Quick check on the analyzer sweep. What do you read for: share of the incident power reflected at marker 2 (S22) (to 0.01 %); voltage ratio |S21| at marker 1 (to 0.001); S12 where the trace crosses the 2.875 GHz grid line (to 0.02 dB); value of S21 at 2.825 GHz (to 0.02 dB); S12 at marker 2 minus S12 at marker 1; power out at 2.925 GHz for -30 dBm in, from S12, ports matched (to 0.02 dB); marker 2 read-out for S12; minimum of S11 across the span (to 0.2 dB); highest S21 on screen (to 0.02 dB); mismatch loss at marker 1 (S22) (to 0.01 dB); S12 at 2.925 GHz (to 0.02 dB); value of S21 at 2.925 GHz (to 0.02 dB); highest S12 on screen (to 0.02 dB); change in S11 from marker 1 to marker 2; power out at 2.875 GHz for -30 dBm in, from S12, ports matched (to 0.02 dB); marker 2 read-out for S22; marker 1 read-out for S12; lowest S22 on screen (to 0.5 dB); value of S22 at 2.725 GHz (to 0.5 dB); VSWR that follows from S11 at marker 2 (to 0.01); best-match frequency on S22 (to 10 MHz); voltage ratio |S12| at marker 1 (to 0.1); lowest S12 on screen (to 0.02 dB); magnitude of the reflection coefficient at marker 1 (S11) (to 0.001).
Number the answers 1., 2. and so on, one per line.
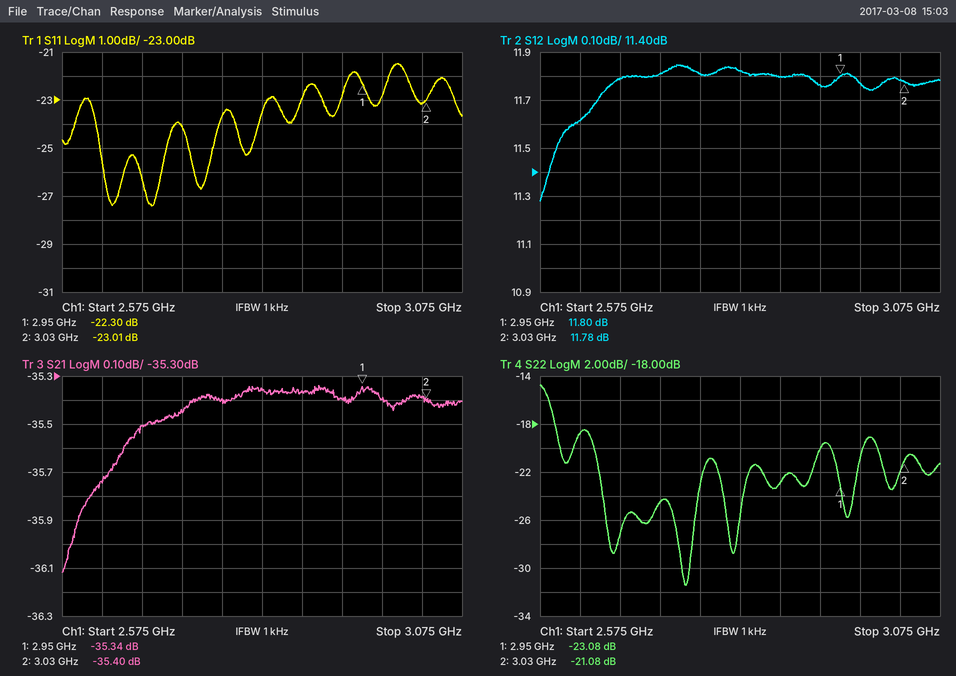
1. 0.78 %
2. 0.017
3. 11.80 dB
4. -35.36 dB
5. -0.02 dB
6. -18.24 dBm
7. 11.78 dB
8. -27.4 dB
9. -35.34 dB
10. 0.02 dB
11. 11.76 dB
12. -35.40 dB
13. 11.84 dB
14. -0.71 dB
15. -18.20 dBm
16. -21.08 dB
17. 11.80 dB
18. -31.5 dB
19. -24.5 dB
20. 1.15
21. 2.76 GHz
22. 3.9
23. 11.28 dB
24. 0.077
